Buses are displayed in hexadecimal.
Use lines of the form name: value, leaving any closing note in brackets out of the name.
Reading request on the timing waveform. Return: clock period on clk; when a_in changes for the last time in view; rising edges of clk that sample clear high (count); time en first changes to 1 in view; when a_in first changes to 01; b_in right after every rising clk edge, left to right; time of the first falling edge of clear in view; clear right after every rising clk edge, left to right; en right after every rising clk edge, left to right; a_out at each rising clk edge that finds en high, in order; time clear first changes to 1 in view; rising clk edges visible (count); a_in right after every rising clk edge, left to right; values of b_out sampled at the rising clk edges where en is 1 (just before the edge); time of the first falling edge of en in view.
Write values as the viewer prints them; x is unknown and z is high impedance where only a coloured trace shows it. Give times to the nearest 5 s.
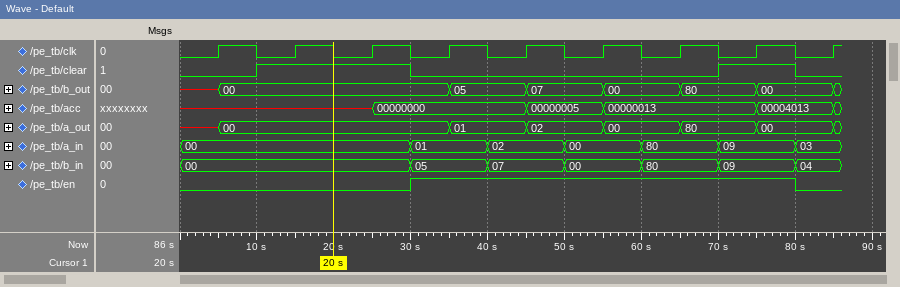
clock period on clk: 10 s
when a_in changes for the last time in view: 80 s
rising edges of clk that sample clear high: 3
time en first changes to 1 in view: 30 s
when a_in first changes to 01: 30 s
b_in right after every rising clk edge, left to right: 00, 00, 00, 05, 07, 00, 80, 09, 04
time of the first falling edge of clear in view: 30 s
clear right after every rising clk edge, left to right: 0 1 1 0 0 0 0 1 0
en right after every rising clk edge, left to right: 0 0 0 1 1 1 1 1 0
a_out at each rising clk edge that finds en high, in order: 00, 01, 02, 00, 80
time clear first changes to 1 in view: 10 s
rising clk edges visible: 9
a_in right after every rising clk edge, left to right: 00, 00, 00, 01, 02, 00, 80, 09, 03
values of b_out sampled at the rising clk edges where en is 1: 00, 05, 07, 00, 80
time of the first falling edge of en in view: 80 s
